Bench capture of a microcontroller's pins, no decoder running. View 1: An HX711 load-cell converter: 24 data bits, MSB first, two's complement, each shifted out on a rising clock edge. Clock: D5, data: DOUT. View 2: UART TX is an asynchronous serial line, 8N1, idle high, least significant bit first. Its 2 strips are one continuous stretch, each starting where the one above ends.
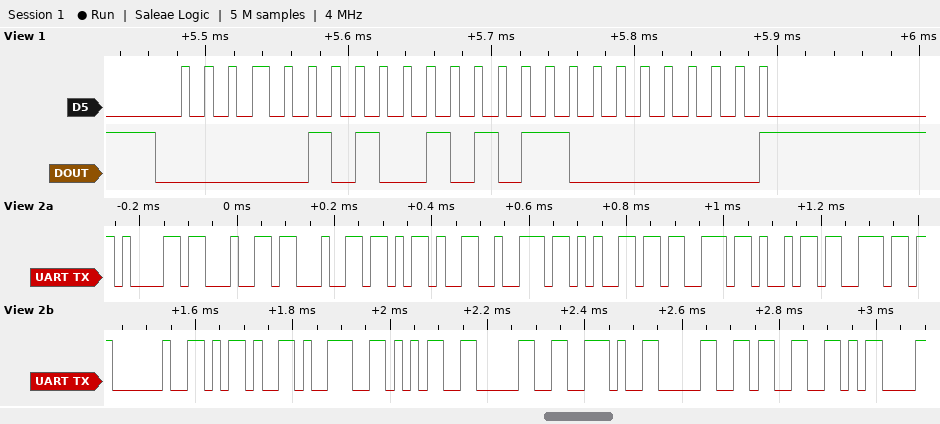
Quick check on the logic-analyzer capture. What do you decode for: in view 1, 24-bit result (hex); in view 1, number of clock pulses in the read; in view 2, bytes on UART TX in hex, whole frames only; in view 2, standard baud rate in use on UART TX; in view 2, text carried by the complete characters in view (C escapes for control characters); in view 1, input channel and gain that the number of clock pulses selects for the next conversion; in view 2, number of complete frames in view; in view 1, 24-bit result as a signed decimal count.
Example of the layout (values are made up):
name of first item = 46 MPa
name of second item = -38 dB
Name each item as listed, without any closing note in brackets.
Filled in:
in view 1, 24-bit result = 0x052B00
in view 1, number of clock pulses in the read = 25
in view 2, bytes on UART TX in hex, whole frames only = 0x61 0x64 0x64 0x2D 0x72 0x65 0x73 0x69 0x6E 0x20 0x2D 0x39 0x35 0x30 0x2E 0x30 0x33 0x0D
in view 2, standard baud rate in use on UART TX = 57600 baud
in view 2, text carried by the complete characters in view = "add-resin -950.03\r"
in view 1, input channel and gain that the number of clock pulses selects for the next conversion = channel A, gain 128
in view 2, number of complete frames in view = 18
in view 1, 24-bit result as a signed decimal count = 338688
